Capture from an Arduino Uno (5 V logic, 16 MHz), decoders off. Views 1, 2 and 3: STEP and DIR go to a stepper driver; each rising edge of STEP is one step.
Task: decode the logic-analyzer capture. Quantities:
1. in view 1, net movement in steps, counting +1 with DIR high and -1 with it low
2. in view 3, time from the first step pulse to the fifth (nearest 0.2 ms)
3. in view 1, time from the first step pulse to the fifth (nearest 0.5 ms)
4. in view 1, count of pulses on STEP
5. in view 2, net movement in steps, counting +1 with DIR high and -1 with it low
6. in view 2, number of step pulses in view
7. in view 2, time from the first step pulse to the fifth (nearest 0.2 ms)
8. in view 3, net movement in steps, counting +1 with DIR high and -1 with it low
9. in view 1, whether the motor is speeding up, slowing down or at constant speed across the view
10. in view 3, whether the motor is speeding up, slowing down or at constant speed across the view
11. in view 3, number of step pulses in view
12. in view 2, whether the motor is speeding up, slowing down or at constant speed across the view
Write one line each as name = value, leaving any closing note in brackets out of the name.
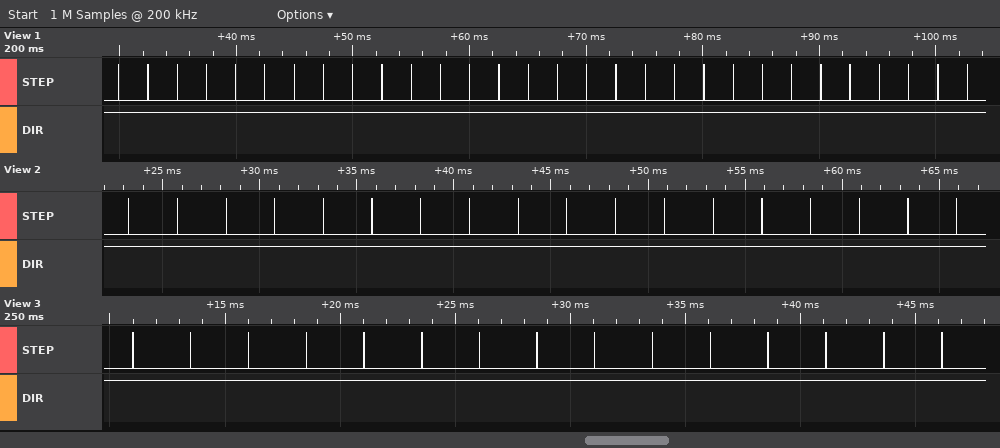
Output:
in view 1, net movement in steps, counting +1 with DIR high and -1 with it low = +30
in view 3, time from the first step pulse to the fifth = 10.0 ms
in view 1, time from the first step pulse to the fifth = 10.0 ms
in view 1, count of pulses on STEP = 30
in view 2, net movement in steps, counting +1 with DIR high and -1 with it low = +18
in view 2, number of step pulses in view = 18
in view 2, time from the first step pulse to the fifth = 10.0 ms
in view 3, net movement in steps, counting +1 with DIR high and -1 with it low = +15
in view 1, whether the motor is speeding up, slowing down or at constant speed across the view = constant speed
in view 3, whether the motor is speeding up, slowing down or at constant speed across the view = constant speed
in view 3, number of step pulses in view = 15
in view 2, whether the motor is speeding up, slowing down or at constant speed across the view = constant speed
